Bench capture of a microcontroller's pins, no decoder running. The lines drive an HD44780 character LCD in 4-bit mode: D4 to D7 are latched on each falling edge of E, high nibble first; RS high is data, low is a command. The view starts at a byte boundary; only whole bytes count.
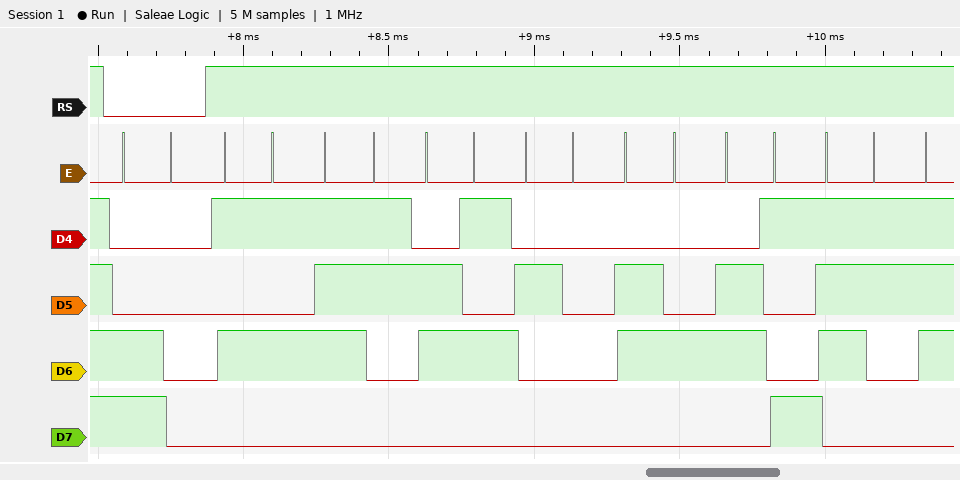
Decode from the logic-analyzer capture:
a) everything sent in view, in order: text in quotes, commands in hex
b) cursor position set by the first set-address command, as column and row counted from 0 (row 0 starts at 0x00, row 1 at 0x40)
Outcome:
0xC0 "Use dis"
column 0, row 1
